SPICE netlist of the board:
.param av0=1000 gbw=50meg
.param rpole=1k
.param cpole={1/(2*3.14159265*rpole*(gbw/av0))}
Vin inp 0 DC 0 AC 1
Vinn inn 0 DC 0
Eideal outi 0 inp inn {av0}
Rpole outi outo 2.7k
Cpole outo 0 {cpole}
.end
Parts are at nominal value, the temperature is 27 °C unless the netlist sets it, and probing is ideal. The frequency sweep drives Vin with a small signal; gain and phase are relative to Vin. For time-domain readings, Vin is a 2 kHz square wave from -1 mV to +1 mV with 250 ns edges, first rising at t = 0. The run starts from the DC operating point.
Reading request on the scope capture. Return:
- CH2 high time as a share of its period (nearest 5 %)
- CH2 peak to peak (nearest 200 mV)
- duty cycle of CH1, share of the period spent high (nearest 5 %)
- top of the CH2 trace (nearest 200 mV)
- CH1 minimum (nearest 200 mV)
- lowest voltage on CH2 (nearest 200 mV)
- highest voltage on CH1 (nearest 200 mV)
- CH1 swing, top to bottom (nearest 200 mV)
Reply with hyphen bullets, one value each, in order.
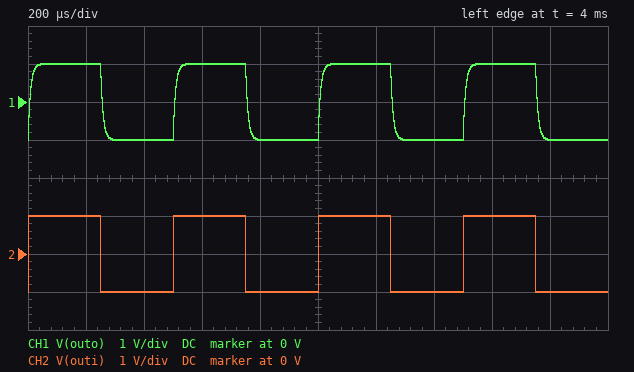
- 50 %
- 2.0 V
- 50 %
- 1.0 V
- -1.0 V
- -1.0 V
- 1.0 V
- 2.0 V
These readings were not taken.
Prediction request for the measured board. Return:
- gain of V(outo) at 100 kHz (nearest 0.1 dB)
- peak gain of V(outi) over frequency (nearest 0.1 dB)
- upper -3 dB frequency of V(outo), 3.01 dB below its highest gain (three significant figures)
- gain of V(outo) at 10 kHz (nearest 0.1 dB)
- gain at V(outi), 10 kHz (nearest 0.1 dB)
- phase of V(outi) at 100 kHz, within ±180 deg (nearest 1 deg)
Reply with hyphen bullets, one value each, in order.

- 45.2 dB
- 60.0 dB
- 18.5 kHz
- 58.9 dB
- 60.0 dB
- 0 deg
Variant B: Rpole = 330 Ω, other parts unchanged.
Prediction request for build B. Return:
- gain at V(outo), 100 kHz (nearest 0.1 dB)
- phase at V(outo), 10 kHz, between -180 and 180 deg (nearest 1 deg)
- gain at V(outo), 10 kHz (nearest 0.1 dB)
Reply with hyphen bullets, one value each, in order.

- 58.4 dB
- -4 deg
- 60.0 dB
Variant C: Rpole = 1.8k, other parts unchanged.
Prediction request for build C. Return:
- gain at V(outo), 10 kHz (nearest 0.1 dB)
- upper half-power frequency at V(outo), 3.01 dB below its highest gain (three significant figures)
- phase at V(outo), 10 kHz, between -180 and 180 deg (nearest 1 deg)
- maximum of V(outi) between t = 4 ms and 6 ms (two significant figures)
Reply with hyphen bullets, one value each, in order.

- 59.5 dB
- 27.8 kHz
- -20 deg
- 1.0 V
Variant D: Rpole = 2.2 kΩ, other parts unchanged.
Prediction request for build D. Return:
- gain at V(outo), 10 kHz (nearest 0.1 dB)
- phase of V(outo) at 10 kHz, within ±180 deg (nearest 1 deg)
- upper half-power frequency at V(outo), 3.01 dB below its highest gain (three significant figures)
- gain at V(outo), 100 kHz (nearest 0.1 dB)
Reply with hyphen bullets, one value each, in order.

- 59.2 dB
- -24 deg
- 22.7 kHz
- 46.9 dB
